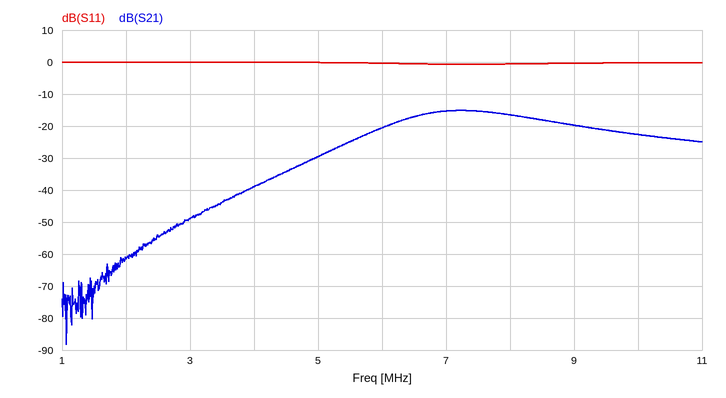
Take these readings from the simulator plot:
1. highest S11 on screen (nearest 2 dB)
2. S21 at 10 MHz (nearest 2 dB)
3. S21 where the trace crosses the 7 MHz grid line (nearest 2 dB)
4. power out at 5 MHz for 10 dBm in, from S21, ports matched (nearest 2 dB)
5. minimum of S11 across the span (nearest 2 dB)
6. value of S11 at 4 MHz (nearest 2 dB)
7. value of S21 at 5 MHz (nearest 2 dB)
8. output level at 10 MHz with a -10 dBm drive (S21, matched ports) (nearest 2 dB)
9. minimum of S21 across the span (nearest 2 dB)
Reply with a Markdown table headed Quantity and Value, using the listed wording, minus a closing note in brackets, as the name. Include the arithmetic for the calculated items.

| Quantity | Value |
|---|---|
| highest S11 on screen | 0 dB |
| S21 at 10 MHz | -22 dB |
| S21 where the trace crosses the 7 MHz grid line | -16 dB |
| power out at 5 MHz for 10 dBm in, from S21, ports matched | 10 dBm + (-30 dB) = -20 dBm |
| minimum of S11 across the span | 0 dB |
| value of S11 at 4 MHz | 0 dB |
| value of S21 at 5 MHz | -30 dB |
| output level at 10 MHz with a -10 dBm drive (S21, matched ports) | -10 dBm + (-22 dB) = -32 dBm |
| minimum of S21 across the span | -88 dB |
